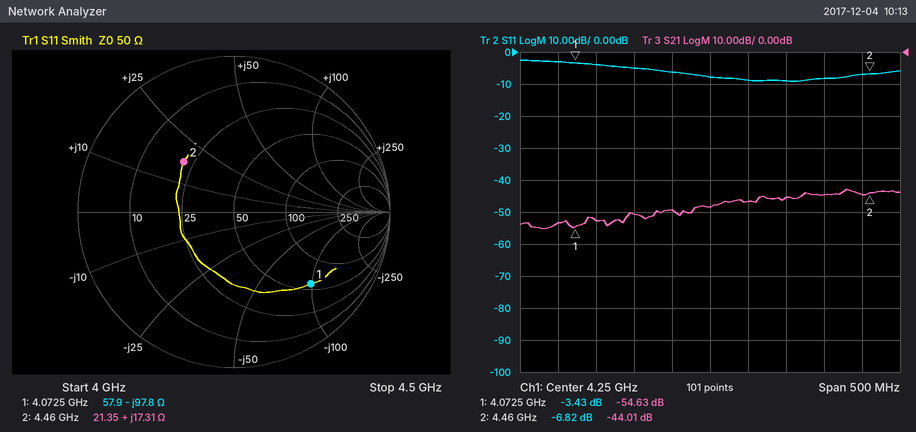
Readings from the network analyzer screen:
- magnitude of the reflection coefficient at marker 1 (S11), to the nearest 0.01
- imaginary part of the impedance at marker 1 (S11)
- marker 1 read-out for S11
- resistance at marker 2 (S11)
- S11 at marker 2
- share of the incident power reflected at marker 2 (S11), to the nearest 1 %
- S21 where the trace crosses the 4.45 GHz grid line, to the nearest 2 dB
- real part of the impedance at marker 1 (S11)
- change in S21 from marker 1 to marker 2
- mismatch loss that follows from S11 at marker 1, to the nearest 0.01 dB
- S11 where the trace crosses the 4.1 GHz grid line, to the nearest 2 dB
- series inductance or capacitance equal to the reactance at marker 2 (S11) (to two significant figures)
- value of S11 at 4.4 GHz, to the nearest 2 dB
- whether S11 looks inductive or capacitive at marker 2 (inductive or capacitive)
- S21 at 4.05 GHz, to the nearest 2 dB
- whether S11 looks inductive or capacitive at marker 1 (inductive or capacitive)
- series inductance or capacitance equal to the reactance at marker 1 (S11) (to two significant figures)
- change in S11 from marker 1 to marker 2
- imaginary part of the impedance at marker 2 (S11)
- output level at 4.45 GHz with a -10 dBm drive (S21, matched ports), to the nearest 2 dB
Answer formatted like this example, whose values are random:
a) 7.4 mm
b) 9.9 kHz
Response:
a) 0.67
b) -97.8 Ω
c) -3.43 dB
d) 21.35 Ω
e) -6.82 dB
f) 21 %
g) -44 dB
h) 57.9 Ω
i) 10.62 dB
j) 2.63 dB
k) -4 dB
l) 620 pH
m) -8 dB
n) inductive
o) -54 dB
p) capacitive
q) 400 fF
r) -3.39 dB
s) +17.31 Ω
t) -54 dBm
